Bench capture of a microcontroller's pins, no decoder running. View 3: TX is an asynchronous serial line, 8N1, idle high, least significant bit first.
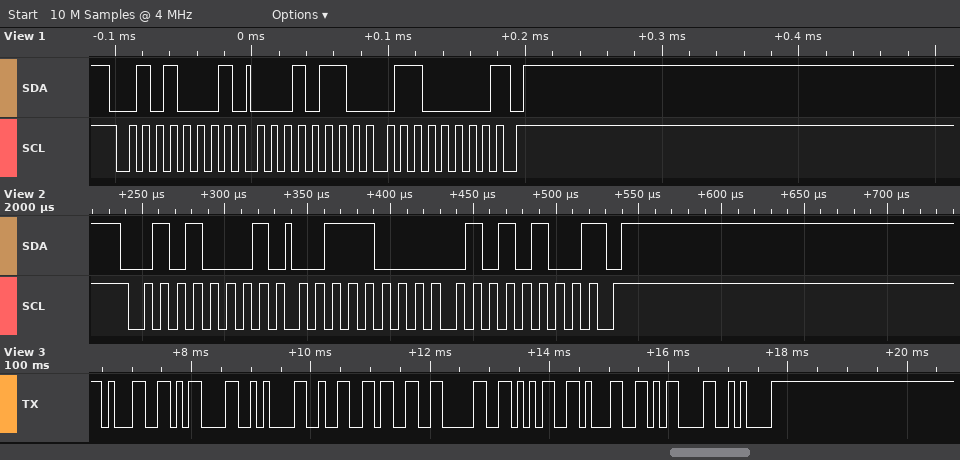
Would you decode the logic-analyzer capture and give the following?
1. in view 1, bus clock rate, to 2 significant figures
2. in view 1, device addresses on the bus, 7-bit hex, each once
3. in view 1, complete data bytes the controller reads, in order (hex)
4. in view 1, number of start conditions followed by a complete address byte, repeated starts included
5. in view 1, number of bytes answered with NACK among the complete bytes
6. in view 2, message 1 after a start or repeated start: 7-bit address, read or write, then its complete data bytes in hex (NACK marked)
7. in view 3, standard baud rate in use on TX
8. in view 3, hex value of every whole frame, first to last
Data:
100 kHz
0x28
16 60
1
1
0x28 read: 38 54 NACK
9600 baud
31 0D 0A 32 33 30 35 31 0D 0A
